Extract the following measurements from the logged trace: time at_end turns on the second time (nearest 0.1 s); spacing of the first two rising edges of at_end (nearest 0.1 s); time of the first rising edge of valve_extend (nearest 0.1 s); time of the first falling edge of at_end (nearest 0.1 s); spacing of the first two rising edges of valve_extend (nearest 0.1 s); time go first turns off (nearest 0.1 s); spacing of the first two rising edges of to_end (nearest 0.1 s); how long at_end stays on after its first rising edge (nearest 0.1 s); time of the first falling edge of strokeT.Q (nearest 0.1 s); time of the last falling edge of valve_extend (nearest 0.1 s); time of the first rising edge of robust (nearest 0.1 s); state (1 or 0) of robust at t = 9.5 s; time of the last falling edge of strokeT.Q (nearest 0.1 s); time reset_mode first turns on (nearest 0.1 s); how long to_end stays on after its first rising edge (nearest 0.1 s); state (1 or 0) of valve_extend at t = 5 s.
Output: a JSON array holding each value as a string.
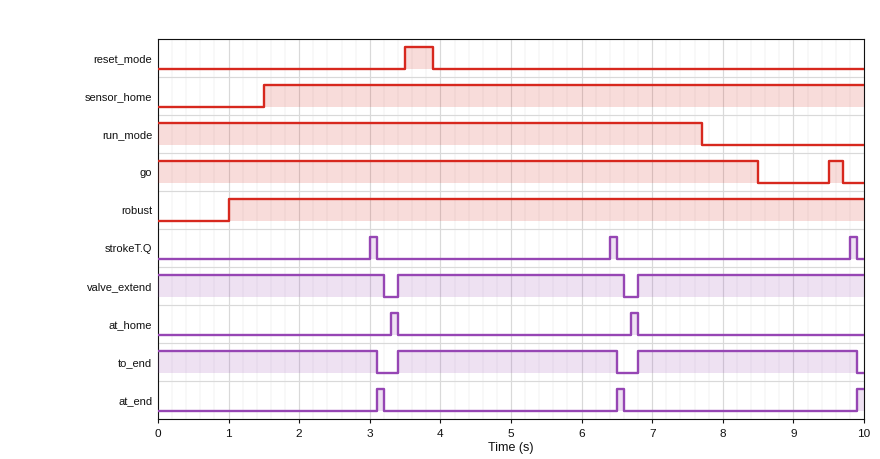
["6.5 s", "3.4 s", "3.4 s", "3.2 s", "3.4 s", "8.5 s", "3.4 s", "0.1 s", "3.1 s", "6.6 s", "1.0 s", "1", "9.9 s", "3.5 s", "3.1 s", "1"]
